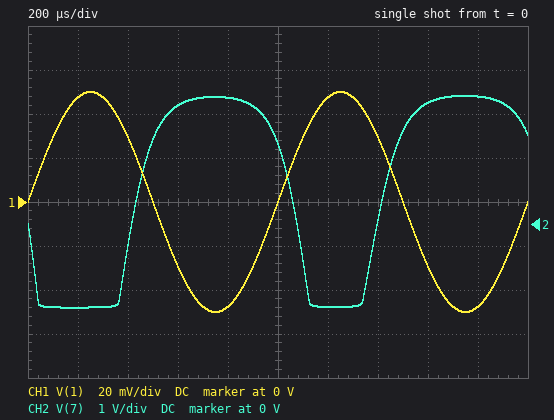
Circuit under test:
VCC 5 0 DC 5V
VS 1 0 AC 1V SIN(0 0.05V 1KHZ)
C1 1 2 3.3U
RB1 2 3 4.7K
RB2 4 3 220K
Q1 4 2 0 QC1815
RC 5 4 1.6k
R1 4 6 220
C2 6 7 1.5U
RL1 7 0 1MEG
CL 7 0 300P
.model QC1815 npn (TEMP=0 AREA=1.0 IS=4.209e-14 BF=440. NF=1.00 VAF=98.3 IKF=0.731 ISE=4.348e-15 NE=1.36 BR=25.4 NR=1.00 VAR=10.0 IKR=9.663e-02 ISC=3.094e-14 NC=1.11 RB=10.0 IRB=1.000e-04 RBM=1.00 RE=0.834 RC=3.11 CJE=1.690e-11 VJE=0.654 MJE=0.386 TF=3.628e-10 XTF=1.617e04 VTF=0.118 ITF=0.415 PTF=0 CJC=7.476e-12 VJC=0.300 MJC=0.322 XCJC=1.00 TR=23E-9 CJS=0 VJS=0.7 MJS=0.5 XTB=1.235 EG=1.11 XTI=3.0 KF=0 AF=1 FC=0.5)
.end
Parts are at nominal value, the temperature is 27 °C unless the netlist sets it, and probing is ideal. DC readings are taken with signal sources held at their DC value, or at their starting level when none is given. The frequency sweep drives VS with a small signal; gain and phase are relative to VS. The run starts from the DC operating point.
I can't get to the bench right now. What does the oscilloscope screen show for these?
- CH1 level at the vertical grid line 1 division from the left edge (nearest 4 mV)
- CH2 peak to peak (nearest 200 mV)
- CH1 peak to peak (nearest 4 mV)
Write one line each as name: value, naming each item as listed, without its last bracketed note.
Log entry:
CH1 level at the vertical grid line 1 division from the left edge: 48 mV
CH2 peak to peak: 4.8 V
CH1 peak to peak: 100 mV
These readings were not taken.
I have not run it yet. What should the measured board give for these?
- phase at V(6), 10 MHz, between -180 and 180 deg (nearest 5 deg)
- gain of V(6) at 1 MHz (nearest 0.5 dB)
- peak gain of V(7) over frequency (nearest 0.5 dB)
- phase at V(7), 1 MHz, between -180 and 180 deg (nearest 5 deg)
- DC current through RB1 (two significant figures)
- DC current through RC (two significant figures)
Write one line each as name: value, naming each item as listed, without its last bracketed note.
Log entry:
phase at V(6), 10 MHz, between -180 and 180 deg: 85 deg
gain of V(6) at 1 MHz: 30.5 dB
peak gain of V(7) over frequency: 41.5 dB
phase at V(7), 1 MHz, between -180 and 180 deg: 105 deg
DC current through RB1: 5.5 µA
DC current through RC: 1.9 mA
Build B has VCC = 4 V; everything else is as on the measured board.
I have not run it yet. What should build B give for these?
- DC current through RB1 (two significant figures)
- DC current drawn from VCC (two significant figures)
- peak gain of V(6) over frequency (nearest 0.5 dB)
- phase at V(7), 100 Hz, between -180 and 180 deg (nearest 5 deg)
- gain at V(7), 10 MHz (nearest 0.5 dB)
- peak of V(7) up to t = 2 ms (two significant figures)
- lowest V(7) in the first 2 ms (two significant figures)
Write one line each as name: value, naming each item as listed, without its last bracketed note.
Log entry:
DC current through RB1: 4.3 µA
DC current drawn from VCC: 1.5 mA
peak gain of V(6) over frequency: 39.0 dB
phase at V(7), 100 Hz, between -180 and 180 deg: -165 deg
gain at V(7), 10 MHz: 8.5 dB
peak of V(7) up to t = 2 ms: 2.2 V
lowest V(7) in the first 2 ms: -1.6 V
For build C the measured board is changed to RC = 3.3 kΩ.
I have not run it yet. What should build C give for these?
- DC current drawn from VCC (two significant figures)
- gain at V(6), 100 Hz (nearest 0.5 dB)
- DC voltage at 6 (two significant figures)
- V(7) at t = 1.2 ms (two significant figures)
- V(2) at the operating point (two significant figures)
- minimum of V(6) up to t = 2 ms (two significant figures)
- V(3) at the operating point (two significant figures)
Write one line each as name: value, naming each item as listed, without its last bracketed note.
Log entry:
DC current drawn from VCC: 1.1 mA
gain at V(6), 100 Hz: 42.5 dB
DC voltage at 6: 1.4 V
V(7) at t = 1.2 ms: -1.4 V
V(2) at the operating point: 670 mV
minimum of V(6) up to t = 2 ms: 19 mV
V(3) at the operating point: 690 mV
